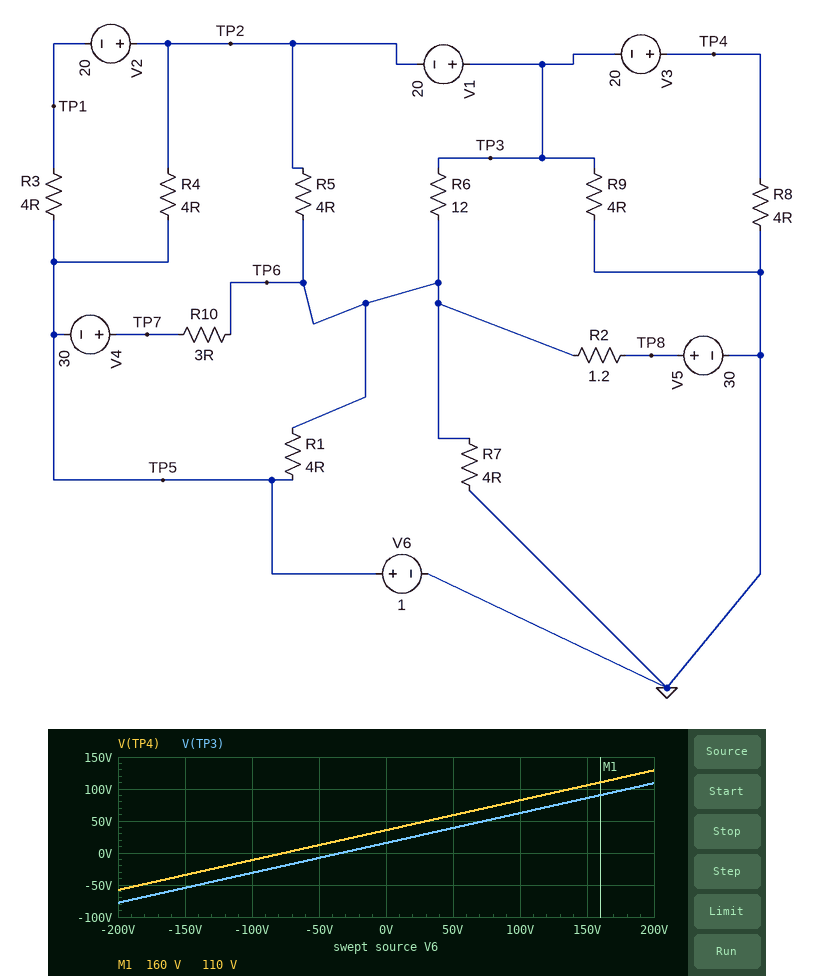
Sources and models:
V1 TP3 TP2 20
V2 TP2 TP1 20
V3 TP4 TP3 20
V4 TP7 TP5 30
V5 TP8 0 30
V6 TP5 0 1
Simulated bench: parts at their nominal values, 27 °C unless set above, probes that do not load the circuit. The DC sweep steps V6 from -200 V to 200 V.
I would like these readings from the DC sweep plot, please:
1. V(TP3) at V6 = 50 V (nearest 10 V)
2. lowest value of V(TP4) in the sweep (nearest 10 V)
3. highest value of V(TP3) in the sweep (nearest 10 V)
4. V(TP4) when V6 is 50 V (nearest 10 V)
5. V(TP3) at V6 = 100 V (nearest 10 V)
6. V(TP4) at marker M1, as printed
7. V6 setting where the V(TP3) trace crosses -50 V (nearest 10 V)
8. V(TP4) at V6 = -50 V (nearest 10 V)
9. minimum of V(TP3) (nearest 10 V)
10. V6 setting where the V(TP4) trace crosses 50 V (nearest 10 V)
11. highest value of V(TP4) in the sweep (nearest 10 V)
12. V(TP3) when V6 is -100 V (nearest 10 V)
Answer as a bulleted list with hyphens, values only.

- 40 V
- -60 V
- 110 V
- 60 V
- 60 V
- 110 V
- -140 V
- 10 V
- -80 V
- 30 V
- 130 V
- -30 V
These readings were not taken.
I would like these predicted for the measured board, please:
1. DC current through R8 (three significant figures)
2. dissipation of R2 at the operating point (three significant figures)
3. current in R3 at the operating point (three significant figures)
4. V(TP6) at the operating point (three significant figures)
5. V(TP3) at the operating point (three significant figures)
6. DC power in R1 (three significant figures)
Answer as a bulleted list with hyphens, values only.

- 9.03 A
- 120 W
- 6.22 A
- 18.0 V
- 16.1 V
- 72.1 W
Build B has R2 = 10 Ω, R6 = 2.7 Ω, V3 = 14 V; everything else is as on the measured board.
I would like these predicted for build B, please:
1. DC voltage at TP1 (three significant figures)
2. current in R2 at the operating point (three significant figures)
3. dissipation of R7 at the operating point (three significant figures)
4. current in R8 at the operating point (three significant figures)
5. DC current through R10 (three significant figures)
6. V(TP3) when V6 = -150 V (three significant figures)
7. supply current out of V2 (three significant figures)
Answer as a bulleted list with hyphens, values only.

- -25.1 V
- 1.85 A
- 32.9 W
- 7.22 A
- 6.51 A
- -65.7 V
- 6.53 A
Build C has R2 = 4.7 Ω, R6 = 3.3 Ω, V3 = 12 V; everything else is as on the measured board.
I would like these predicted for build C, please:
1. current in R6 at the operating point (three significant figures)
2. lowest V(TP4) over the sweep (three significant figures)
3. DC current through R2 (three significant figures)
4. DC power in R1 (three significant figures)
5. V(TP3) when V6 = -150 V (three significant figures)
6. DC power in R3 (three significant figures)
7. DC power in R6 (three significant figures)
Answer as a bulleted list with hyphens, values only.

- 882 mA
- -75.7 V
- 3.62 A
- 35.9 W
- -61.9 V
- 158 W
- 2.57 W
